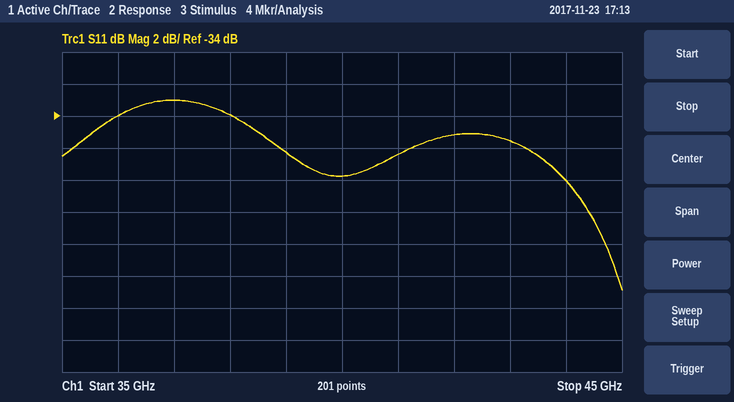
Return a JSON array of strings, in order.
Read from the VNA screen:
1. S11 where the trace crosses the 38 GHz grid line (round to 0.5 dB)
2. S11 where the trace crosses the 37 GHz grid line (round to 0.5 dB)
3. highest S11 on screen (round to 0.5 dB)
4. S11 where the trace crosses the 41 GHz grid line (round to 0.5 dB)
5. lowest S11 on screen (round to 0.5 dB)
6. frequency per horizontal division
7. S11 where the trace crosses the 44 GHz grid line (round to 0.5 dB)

["-34.0 dB", "-33.0 dB", "-33.0 dB", "-36.5 dB", "-45.0 dB", "1 GHz", "-38.0 dB"]
